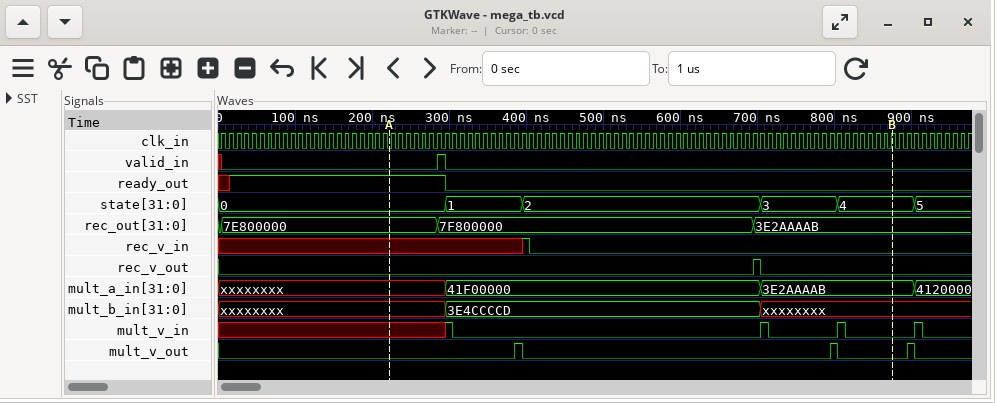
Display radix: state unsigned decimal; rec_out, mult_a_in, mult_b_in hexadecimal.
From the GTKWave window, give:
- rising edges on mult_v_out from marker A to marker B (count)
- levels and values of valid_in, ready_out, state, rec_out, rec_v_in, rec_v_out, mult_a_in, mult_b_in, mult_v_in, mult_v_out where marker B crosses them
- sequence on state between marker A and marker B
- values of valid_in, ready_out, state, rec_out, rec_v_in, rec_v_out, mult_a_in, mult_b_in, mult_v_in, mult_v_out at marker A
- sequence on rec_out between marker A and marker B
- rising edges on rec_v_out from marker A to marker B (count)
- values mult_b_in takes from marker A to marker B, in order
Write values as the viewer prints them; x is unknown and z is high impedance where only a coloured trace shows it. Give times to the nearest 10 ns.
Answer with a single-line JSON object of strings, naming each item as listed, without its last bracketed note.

{"rising edges on mult_v_out from marker A to marker B": "2", "levels and values of valid_in, ready_out, state, rec_out, rec_v_in, rec_v_out, mult_a_in, mult_b_in, mult_v_in, mult_v_out where marker B crosses them": "valid_in=0, ready_out=0, state=4, rec_out=3E2AAAAB, rec_v_in=0, rec_v_out=0, mult_a_in=3E2AAAAB, mult_b_in=xxxxxxxx, mult_v_in=0, mult_v_out=0", "sequence on state between marker A and marker B": "0, 1, 2, 3, 4", "values of valid_in, ready_out, state, rec_out, rec_v_in, rec_v_out, mult_a_in, mult_b_in, mult_v_in, mult_v_out at marker A": "valid_in=0, ready_out=1, state=0, rec_out=7E800000, rec_v_in=x, rec_v_out=0, mult_a_in=xxxxxxxx, mult_b_in=xxxxxxxx, mult_v_in=x, mult_v_out=0", "sequence on rec_out between marker A and marker B": "7E800000, 7F800000, 3E2AAAAB", "rising edges on rec_v_out from marker A to marker B": "1", "values mult_b_in takes from marker A to marker B, in order": "xxxxxxxx, 3E4CCCCD, xxxxxxxx"}
